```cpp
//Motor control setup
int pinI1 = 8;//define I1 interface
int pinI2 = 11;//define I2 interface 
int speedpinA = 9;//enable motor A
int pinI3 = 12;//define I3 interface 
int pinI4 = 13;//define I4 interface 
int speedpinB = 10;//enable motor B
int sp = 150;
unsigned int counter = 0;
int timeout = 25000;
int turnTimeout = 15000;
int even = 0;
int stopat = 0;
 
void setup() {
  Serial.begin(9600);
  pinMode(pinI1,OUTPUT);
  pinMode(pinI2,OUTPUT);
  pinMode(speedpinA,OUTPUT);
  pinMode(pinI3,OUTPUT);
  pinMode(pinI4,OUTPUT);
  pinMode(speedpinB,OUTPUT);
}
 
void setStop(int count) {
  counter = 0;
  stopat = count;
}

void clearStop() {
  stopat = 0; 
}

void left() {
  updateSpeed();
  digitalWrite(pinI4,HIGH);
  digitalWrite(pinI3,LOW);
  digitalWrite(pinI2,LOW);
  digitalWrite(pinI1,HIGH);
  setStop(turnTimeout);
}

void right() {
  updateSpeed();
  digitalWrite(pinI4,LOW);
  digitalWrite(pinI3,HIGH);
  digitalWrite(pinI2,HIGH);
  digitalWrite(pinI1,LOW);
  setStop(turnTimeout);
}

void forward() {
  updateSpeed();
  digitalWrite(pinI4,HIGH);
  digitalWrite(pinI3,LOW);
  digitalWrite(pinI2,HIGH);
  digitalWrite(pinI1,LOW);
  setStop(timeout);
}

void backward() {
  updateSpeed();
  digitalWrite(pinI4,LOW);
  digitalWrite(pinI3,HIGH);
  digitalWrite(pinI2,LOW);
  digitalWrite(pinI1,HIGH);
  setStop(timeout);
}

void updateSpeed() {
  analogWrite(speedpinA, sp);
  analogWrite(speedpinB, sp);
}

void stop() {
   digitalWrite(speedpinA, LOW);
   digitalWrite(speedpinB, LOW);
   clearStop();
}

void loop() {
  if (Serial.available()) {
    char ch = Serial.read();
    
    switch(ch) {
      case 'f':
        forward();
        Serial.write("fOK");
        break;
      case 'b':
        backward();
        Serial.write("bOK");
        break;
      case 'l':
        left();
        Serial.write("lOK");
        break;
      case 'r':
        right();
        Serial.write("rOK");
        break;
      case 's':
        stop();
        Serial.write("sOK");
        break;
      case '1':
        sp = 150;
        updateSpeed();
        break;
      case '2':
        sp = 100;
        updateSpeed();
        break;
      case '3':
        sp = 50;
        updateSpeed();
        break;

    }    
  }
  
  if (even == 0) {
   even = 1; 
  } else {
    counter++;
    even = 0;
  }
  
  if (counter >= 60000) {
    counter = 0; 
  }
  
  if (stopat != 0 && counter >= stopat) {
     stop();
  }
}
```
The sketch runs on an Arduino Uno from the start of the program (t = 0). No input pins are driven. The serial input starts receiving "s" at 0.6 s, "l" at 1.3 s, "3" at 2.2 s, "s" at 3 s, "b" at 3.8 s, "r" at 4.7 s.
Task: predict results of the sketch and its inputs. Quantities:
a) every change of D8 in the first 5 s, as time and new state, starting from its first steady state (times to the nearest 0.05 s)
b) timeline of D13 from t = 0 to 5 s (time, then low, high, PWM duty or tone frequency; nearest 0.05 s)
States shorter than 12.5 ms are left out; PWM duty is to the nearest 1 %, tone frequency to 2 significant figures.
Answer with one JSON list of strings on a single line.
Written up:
["0 s low; 1.3 s high; 4.7 s low", "0 s low; 1.3 s high; 3.8 s low"]
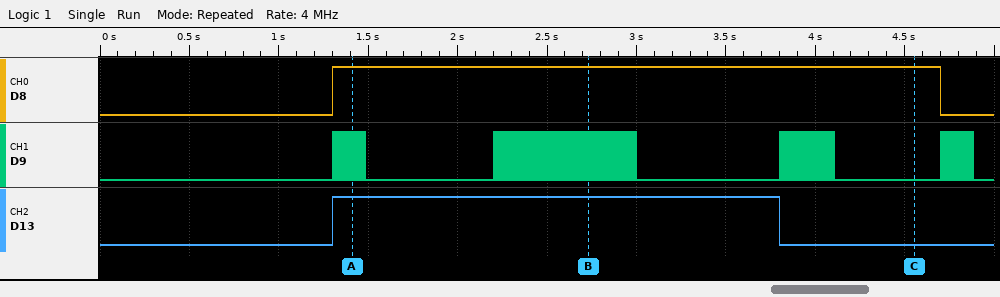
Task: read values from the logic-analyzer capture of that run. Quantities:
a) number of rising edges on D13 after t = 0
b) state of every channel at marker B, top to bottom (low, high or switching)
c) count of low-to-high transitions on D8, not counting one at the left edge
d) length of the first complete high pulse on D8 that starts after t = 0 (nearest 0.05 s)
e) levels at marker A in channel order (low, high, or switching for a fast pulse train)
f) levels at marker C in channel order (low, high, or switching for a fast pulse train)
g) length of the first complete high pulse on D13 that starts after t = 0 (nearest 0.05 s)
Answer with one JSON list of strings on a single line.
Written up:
["1", "D8 high, D9 switching, D13 high", "1", "3.40 s", "D8 high, D9 switching, D13 high", "D8 high, D9 low, D13 low", "2.50 s"]
